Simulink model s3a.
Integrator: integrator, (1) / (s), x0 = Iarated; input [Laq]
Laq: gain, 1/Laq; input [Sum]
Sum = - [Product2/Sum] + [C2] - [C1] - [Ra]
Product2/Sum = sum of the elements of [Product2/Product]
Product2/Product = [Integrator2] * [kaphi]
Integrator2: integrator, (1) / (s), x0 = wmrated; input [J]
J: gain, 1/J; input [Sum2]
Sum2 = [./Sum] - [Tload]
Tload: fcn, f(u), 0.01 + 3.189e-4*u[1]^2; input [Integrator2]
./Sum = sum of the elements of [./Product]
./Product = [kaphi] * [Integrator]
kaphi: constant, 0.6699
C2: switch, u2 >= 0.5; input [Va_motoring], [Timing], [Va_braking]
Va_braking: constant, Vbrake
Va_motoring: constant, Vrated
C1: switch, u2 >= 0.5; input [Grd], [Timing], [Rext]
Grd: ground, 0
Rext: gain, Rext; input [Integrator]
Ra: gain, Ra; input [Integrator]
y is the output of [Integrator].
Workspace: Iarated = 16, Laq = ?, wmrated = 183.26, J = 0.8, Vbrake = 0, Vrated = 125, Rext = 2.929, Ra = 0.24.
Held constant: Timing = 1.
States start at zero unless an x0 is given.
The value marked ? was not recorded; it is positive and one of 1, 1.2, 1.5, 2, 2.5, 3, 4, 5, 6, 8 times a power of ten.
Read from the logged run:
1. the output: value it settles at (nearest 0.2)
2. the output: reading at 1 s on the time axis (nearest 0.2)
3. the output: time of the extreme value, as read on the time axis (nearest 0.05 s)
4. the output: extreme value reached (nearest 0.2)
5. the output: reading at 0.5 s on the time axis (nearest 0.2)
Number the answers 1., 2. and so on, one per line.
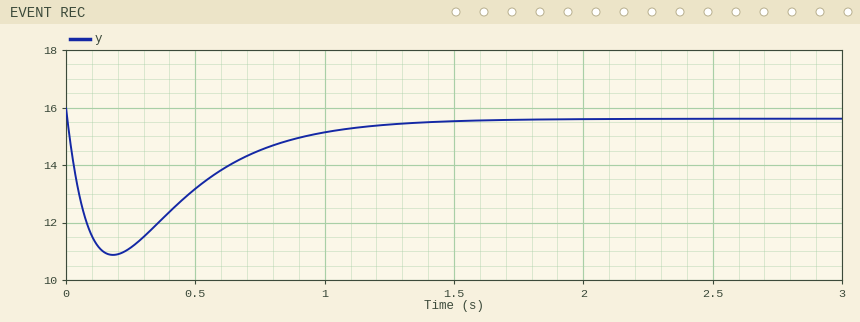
1. 15.6
2. 15.2
3. 0.20 s
4. 10.8
5. 13.2
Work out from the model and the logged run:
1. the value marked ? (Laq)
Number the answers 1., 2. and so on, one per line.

1. 0.02
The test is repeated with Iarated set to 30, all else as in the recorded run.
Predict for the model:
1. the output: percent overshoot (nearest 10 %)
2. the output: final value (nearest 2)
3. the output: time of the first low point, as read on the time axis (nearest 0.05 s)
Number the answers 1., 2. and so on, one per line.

1. 40 %
2. 16
3. 0.25 s
